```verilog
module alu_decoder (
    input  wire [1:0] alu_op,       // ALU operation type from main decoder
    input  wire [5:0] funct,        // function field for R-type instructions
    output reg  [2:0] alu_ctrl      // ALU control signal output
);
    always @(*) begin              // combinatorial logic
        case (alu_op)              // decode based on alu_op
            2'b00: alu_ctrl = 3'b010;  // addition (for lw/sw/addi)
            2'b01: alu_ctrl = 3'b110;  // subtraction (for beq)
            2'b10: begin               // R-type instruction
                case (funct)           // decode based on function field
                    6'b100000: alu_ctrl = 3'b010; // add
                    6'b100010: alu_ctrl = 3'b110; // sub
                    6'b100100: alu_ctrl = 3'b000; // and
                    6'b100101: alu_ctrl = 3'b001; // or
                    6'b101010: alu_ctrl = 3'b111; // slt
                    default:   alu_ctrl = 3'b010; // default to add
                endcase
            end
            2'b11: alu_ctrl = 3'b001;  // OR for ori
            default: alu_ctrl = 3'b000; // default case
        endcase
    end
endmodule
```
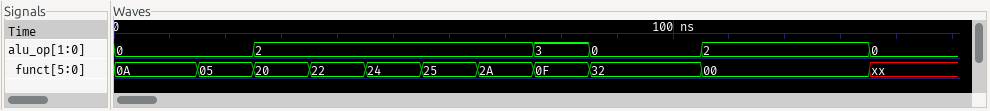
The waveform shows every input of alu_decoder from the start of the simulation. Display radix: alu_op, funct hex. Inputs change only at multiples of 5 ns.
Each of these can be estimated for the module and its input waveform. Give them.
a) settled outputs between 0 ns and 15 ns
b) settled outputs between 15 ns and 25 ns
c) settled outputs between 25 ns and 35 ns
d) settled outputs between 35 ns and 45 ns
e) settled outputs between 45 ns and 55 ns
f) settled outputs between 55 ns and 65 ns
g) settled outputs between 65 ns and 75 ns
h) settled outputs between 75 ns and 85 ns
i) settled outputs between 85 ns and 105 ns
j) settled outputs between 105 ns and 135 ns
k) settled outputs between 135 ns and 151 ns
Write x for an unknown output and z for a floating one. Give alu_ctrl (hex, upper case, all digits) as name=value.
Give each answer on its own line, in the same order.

alu_ctrl=2
alu_ctrl=2
alu_ctrl=2
alu_ctrl=6
alu_ctrl=0
alu_ctrl=1
alu_ctrl=7
alu_ctrl=1
alu_ctrl=2
alu_ctrl=2
alu_ctrl=2
